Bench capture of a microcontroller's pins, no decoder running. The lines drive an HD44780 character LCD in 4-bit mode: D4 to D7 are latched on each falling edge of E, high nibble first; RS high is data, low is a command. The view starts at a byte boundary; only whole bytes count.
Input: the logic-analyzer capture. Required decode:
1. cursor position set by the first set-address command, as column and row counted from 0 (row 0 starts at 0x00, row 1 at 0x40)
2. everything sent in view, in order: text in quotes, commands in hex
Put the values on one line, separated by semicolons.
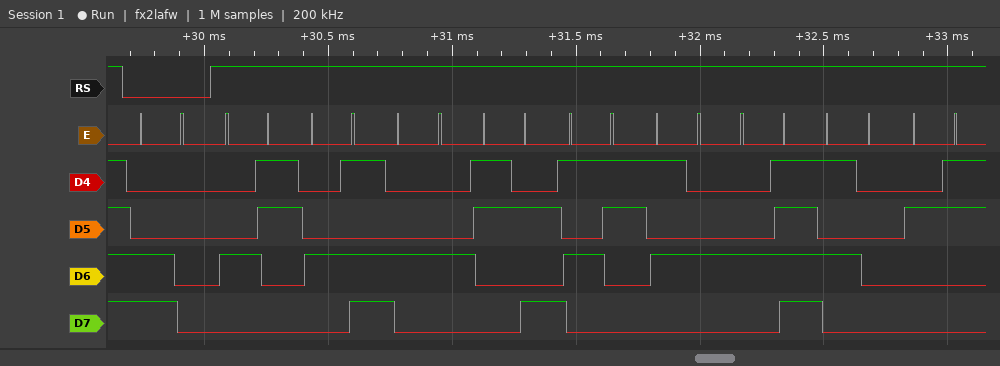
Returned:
column 0, row 1; 0xC0 "CMD:STOP#"
